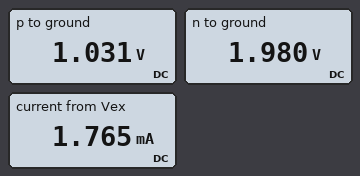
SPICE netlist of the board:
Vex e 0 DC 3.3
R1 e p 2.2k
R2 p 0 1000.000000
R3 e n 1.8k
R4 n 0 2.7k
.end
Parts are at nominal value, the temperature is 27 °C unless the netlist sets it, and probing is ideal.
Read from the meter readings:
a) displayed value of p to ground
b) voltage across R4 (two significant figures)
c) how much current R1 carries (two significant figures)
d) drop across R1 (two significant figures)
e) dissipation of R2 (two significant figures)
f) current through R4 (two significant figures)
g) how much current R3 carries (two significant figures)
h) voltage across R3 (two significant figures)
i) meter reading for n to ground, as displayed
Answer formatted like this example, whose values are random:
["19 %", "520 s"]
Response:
["1.031 V", "2.0 V", "1.0 mA", "2.3 V", "1.1 mW", "730 µA", "730 µA", "1.3 V", "1.980 V"]
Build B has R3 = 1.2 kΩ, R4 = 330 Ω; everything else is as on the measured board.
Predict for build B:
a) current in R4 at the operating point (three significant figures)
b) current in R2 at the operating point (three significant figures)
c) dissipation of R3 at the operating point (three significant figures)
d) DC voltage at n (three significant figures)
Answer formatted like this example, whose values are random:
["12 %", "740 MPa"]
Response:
["2.16 mA", "1.03 mA", "5.58 mW", "712 mV"]
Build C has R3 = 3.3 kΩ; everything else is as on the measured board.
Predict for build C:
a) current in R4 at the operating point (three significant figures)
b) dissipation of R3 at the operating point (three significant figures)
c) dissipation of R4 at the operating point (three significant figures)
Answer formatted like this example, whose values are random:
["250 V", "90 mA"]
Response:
["550 µA", "998 µW", "817 µW"]
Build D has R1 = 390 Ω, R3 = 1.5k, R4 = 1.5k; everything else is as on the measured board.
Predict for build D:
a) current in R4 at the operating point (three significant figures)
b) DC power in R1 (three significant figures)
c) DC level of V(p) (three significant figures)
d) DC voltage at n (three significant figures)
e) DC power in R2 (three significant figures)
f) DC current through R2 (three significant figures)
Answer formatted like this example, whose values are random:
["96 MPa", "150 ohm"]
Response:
["1.10 mA", "2.20 mW", "2.37 V", "1.65 V", "5.64 mW", "2.37 mA"]
